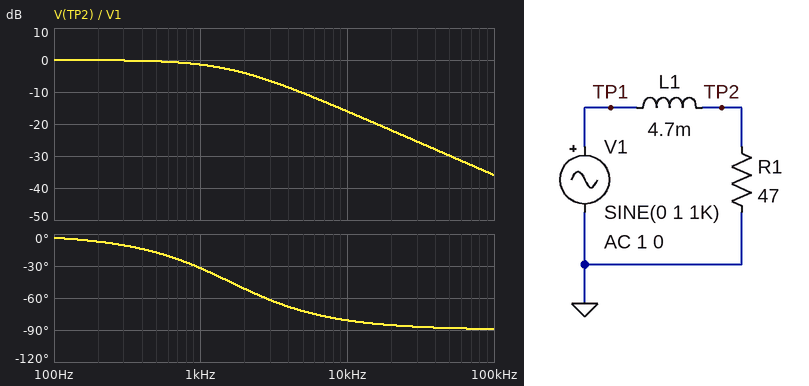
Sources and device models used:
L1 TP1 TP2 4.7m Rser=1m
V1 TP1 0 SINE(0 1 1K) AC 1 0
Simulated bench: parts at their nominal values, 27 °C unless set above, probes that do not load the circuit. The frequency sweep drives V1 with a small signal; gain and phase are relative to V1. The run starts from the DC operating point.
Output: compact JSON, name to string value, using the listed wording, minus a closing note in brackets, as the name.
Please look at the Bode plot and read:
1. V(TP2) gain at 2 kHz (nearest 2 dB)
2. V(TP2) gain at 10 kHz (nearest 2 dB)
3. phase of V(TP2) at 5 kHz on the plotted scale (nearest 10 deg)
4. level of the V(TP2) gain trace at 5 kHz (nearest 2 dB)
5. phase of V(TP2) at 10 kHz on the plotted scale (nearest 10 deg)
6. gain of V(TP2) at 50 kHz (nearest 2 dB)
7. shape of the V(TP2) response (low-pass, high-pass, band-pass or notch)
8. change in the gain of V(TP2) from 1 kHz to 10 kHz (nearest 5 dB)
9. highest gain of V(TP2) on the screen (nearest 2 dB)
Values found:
{"V(TP2) gain at 2 kHz": "-4 dB", "V(TP2) gain at 10 kHz": "-16 dB", "phase of V(TP2) at 5 kHz on the plotted scale": "-70 deg", "level of the V(TP2) gain trace at 5 kHz": "-10 dB", "phase of V(TP2) at 10 kHz on the plotted scale": "-80 deg", "gain of V(TP2) at 50 kHz": "-30 dB", "shape of the V(TP2) response": "low-pass", "change in the gain of V(TP2) from 1 kHz to 10 kHz": "-15 dB", "highest gain of V(TP2) on the screen": "0 dB"}
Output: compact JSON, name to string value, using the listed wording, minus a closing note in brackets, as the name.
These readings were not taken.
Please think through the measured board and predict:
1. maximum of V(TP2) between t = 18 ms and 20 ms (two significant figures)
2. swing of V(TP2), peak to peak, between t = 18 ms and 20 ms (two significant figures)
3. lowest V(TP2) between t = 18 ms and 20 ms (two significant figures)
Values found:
{"maximum of V(TP2) between t = 18 ms and 20 ms": "850 mV", "swing of V(TP2), peak to peak, between t = 18 ms and 20 ms": "1.7 V", "lowest V(TP2) between t = 18 ms and 20 ms": "-850 mV"}
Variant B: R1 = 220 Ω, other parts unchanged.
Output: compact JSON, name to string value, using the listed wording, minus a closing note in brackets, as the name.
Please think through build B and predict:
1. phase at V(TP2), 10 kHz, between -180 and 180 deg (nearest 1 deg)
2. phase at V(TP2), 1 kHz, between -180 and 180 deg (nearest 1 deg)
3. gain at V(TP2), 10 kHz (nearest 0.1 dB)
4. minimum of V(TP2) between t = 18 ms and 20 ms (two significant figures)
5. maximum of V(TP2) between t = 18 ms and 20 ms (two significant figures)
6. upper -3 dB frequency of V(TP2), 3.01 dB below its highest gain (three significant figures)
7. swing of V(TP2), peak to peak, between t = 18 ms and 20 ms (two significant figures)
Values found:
{"phase at V(TP2), 10 kHz, between -180 and 180 deg": "-53 deg", "phase at V(TP2), 1 kHz, between -180 and 180 deg": "-8 deg", "gain at V(TP2), 10 kHz": "-4.5 dB", "minimum of V(TP2) between t = 18 ms and 20 ms": "-990 mV", "maximum of V(TP2) between t = 18 ms and 20 ms": "990 mV", "upper -3 dB frequency of V(TP2), 3.01 dB below its highest gain": "7.45 kHz", "swing of V(TP2), peak to peak, between t = 18 ms and 20 ms": "2.0 V"}
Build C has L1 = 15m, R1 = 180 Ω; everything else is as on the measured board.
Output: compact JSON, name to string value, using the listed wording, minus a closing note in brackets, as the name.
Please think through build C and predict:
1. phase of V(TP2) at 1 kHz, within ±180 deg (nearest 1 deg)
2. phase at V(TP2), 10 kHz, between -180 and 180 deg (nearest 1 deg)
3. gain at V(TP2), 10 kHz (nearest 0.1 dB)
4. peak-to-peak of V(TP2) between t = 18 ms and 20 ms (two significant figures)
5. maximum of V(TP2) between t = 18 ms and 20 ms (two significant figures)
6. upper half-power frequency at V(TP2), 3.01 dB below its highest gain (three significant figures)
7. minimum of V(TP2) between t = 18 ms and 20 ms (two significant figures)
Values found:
{"phase of V(TP2) at 1 kHz, within ±180 deg": "-28 deg", "phase at V(TP2), 10 kHz, between -180 and 180 deg": "-79 deg", "gain at V(TP2), 10 kHz": "-14.5 dB", "peak-to-peak of V(TP2) between t = 18 ms and 20 ms": "1.8 V", "maximum of V(TP2) between t = 18 ms and 20 ms": "890 mV", "upper half-power frequency at V(TP2), 3.01 dB below its highest gain": "1.91 kHz", "minimum of V(TP2) between t = 18 ms and 20 ms": "-890 mV"}
